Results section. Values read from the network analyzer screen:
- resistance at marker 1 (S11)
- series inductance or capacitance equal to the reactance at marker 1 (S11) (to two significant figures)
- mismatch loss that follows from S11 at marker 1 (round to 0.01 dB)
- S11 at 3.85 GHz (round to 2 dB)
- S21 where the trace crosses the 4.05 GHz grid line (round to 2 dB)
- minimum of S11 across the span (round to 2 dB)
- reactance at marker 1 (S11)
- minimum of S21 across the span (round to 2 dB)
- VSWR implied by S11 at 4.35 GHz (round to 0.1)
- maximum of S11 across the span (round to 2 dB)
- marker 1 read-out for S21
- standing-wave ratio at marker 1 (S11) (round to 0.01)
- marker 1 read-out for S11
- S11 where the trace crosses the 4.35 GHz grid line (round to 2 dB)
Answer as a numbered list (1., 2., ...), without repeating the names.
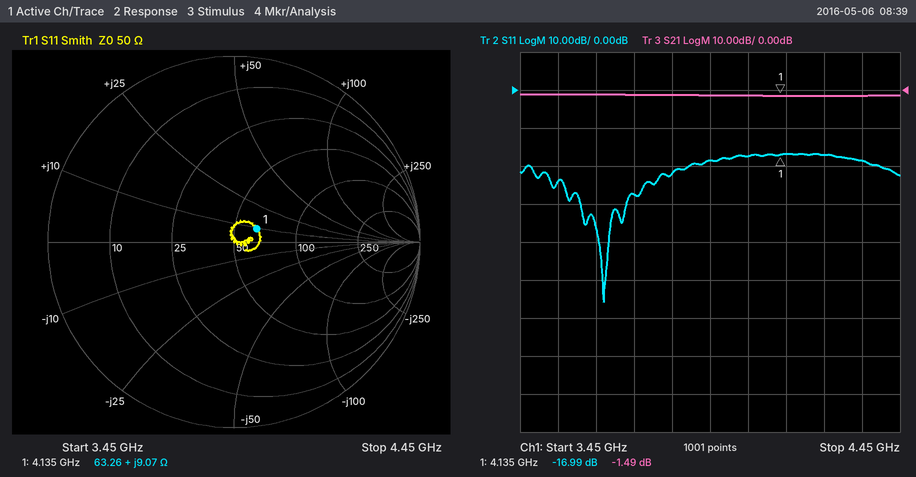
1. 63.26 Ω
2. 350 pH
3. 0.09 dB
4. -22 dB
5. -2 dB
6. -56 dB
7. +9.07 Ω
8. -2 dB
9. 1.3
10. -16 dB
11. -1.49 dB
12. 1.33
13. -16.99 dB
14. -18 dB
